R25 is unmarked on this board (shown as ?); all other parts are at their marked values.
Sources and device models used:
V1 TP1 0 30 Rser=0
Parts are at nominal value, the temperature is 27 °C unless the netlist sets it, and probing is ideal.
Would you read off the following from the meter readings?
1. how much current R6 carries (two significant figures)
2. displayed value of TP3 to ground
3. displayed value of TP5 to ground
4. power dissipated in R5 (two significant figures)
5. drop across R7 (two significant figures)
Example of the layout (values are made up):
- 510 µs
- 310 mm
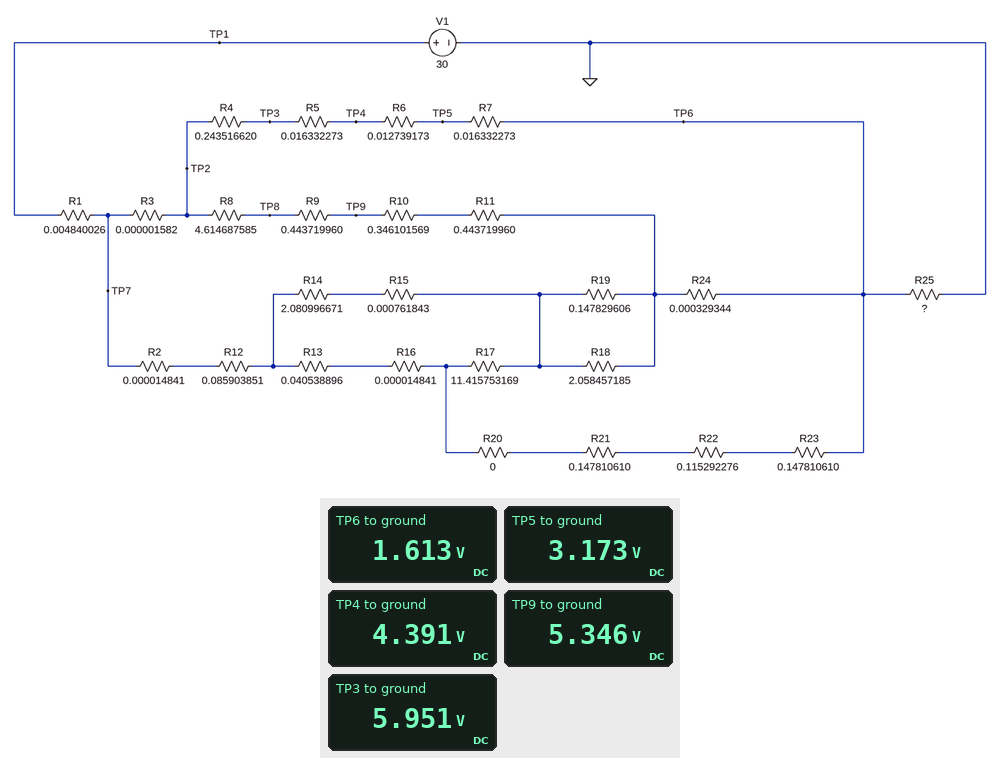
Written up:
- 96 A
- 5.951 V
- 3.173 V
- 150 W
- 1.6 V
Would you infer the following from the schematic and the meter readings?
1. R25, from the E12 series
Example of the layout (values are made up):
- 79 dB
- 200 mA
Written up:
- 0.01 Ω
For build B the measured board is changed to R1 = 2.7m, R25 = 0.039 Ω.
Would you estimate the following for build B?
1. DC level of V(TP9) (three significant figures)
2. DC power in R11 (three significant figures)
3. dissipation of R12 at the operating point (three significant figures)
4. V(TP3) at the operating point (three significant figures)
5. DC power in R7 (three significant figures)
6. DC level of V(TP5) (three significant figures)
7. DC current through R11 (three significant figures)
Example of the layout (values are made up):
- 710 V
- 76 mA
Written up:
- 8.76 V
- 7.55 W
- 244 W
- 9.29 V
- 114 W
- 6.86 V
- 4.12 A
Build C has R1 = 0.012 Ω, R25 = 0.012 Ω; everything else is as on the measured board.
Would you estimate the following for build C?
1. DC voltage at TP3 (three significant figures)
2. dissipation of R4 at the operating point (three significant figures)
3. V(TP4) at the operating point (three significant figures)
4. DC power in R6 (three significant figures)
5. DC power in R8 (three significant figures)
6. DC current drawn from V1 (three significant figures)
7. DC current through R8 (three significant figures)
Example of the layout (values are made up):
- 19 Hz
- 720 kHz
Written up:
- 5.98 V
- 2.02 kW
- 4.49 V
- 106 W
- 93.4 W
- 154 A
- 4.50 A
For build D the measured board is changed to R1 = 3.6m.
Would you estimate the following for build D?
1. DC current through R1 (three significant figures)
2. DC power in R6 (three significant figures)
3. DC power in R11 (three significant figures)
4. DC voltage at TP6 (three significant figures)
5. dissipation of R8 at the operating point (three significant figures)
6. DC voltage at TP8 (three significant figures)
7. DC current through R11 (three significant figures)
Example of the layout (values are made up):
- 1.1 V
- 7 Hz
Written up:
- 162 A
- 118 W
- 10.0 W
- 1.62 V
- 104 W
- 7.49 V
- 4.75 A
